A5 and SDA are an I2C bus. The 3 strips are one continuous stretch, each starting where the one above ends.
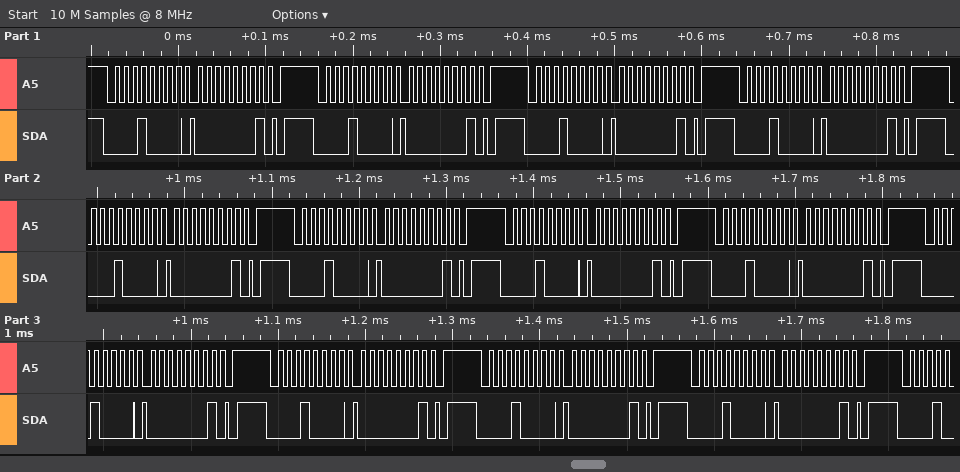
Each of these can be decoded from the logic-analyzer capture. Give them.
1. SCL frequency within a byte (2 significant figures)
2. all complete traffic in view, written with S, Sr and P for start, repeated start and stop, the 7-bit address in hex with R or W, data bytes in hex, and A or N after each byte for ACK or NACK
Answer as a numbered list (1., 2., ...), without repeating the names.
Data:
1. 100 kHz
2. S 08W A 01 A P S 08W A 01 A P S 08W A 01 A P S 08W A 01 A P S 08W A 01 A P S 08W A 01 A P S 08W A 01 A P S 08W A 01 A P S 08W A 01 A P S 08W A 01 A P S 08W A 01 A P S 08W A 01 A P
